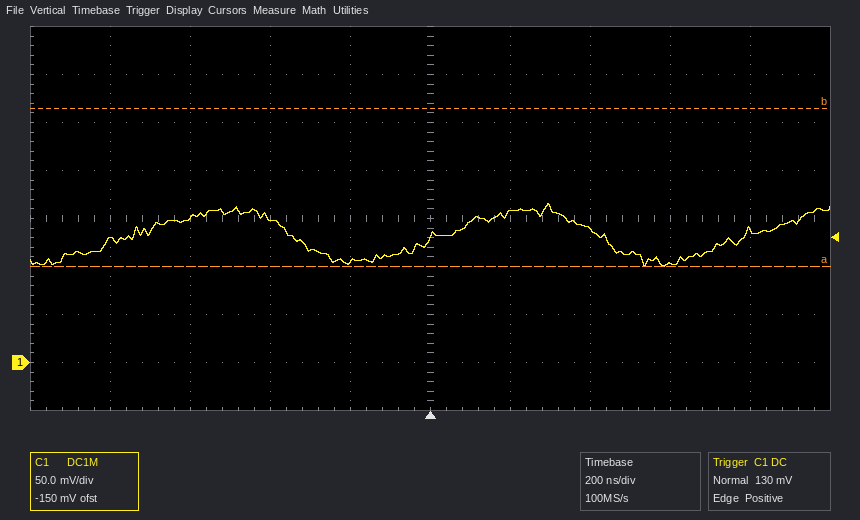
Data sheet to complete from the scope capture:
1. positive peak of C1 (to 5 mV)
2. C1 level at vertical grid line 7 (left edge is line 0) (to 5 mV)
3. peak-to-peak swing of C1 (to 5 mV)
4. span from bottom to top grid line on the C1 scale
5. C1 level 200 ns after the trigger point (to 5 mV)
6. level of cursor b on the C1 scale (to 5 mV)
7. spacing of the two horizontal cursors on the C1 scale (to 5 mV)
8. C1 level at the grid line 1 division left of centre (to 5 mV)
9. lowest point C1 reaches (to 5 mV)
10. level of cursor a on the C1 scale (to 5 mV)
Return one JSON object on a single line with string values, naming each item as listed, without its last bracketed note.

{"positive peak of C1": "165 mV", "C1 level at vertical grid line 7 (left edge is line 0)": "140 mV", "peak-to-peak swing of C1": "65 mV", "span from bottom to top grid line on the C1 scale": "400 mV", "C1 level 200 ns after the trigger point": "155 mV", "level of cursor b on the C1 scale": "265 mV", "spacing of the two horizontal cursors on the C1 scale": "165 mV", "C1 level at the grid line 1 division left of centre": "105 mV", "lowest point C1 reaches": "100 mV", "level of cursor a on the C1 scale": "100 mV"}
